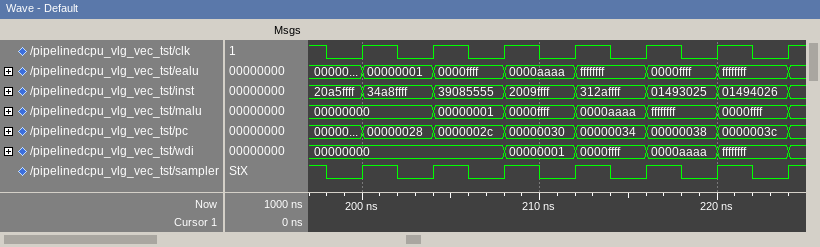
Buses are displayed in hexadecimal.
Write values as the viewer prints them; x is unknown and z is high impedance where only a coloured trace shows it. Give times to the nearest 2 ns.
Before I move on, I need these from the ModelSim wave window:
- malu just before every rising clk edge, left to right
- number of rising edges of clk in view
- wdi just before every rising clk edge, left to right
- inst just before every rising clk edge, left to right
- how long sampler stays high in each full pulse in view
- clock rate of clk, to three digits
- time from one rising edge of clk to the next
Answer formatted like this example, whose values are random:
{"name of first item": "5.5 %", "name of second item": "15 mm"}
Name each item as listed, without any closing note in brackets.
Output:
{"malu just before every rising clk edge, left to right": "00000000, 00000000, 00000001, 0000ffff, 0000aaaa, ffffffff, 0000ffff", "number of rising edges of clk in view": "7", "wdi just before every rising clk edge, left to right": "00000000, 00000000, 00000000, 00000001, 0000ffff, 0000aaaa, ffffffff", "inst just before every rising clk edge, left to right": "20a5ffff, 34a8ffff, 39085555, 2009ffff, 312affff, 01493025, 01494026", "how long sampler stays high in each full pulse in view": "2 ns, 2 ns, 2 ns, 2 ns, 2 ns, 2 ns", "clock rate of clk, to three digits": "250 MHz", "time from one rising edge of clk to the next": "4 ns"}
